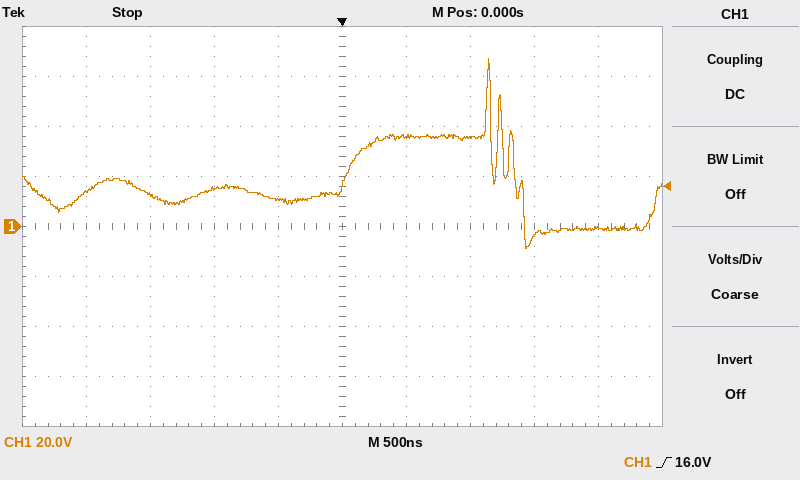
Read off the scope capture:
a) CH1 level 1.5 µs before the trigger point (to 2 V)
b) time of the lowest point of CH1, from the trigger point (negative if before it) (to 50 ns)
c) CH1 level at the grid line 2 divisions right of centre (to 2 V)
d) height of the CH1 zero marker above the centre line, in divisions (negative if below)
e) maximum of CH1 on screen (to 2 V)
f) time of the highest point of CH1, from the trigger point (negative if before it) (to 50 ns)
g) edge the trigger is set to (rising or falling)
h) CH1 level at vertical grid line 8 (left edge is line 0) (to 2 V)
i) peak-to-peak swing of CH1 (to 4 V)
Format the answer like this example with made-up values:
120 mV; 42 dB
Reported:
12 V; +1.45 µs; 36 V; 0.0 div; 68 V; +1.15 µs; rising; -4 V; 76 V
